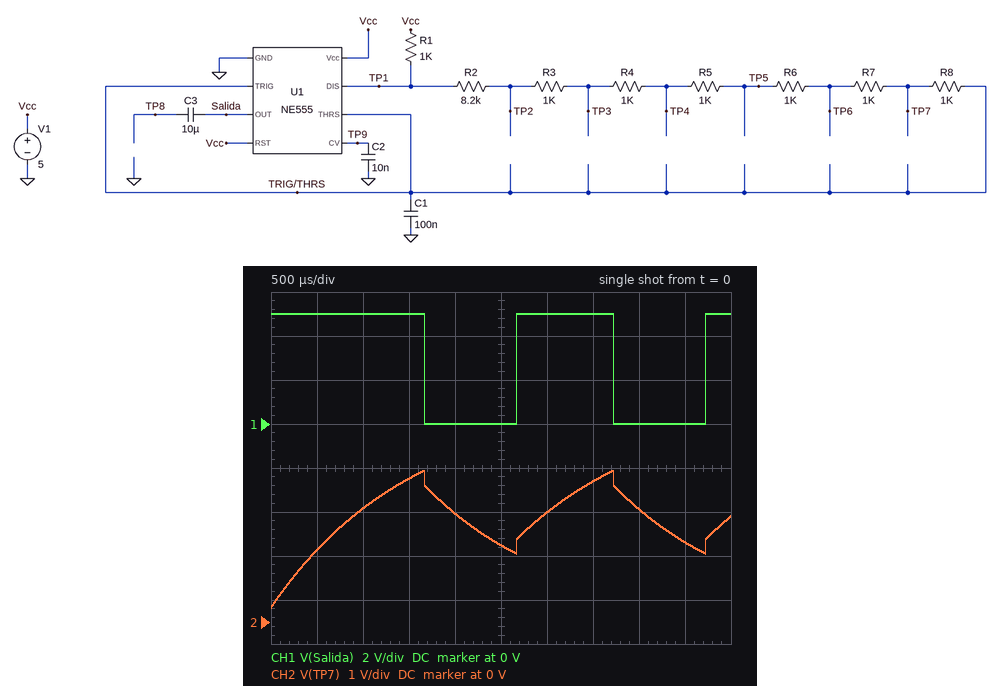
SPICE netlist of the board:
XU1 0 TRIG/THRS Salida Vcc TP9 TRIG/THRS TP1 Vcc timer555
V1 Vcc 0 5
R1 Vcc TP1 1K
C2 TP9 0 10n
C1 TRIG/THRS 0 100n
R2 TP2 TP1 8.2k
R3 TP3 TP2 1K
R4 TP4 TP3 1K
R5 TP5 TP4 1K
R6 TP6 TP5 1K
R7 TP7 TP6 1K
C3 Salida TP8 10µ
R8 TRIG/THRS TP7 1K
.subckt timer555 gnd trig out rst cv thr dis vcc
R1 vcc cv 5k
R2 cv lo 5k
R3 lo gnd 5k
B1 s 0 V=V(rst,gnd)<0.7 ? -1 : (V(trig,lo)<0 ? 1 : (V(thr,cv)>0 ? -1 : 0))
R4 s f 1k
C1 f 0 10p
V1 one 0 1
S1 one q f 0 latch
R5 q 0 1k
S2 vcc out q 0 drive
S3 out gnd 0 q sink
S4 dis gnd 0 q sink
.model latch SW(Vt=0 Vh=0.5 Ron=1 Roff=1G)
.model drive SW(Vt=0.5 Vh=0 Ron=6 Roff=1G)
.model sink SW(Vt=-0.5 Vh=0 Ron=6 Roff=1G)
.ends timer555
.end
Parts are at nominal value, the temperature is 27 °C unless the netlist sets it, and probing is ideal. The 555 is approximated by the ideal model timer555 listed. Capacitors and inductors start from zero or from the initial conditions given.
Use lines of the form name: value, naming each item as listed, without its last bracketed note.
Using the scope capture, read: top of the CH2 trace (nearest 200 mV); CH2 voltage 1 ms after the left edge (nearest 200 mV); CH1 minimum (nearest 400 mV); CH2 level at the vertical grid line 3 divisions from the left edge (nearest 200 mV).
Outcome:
top of the CH2 trace: 3.4 V
CH2 voltage 1 ms after the left edge: 2.6 V
CH1 minimum: 0 V
CH2 level at the vertical grid line 3 divisions from the left edge: 3.2 V
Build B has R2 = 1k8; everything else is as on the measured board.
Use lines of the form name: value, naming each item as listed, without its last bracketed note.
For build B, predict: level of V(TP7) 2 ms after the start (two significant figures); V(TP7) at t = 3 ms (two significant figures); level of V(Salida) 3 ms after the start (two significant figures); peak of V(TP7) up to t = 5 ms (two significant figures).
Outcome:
level of V(TP7) 2 ms after the start: 3.3 V
V(TP7) at t = 3 ms: 3.0 V
level of V(Salida) 3 ms after the start: 5.0 V
peak of V(TP7) up to t = 5 ms: 3.5 V
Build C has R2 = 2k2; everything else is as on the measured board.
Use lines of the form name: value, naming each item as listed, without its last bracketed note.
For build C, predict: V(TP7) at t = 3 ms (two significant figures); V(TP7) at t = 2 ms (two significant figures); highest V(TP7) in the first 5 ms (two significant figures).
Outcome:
V(TP7) at t = 3 ms: 2.6 V
V(TP7) at t = 2 ms: 3.1 V
highest V(TP7) in the first 5 ms: 3.5 V
